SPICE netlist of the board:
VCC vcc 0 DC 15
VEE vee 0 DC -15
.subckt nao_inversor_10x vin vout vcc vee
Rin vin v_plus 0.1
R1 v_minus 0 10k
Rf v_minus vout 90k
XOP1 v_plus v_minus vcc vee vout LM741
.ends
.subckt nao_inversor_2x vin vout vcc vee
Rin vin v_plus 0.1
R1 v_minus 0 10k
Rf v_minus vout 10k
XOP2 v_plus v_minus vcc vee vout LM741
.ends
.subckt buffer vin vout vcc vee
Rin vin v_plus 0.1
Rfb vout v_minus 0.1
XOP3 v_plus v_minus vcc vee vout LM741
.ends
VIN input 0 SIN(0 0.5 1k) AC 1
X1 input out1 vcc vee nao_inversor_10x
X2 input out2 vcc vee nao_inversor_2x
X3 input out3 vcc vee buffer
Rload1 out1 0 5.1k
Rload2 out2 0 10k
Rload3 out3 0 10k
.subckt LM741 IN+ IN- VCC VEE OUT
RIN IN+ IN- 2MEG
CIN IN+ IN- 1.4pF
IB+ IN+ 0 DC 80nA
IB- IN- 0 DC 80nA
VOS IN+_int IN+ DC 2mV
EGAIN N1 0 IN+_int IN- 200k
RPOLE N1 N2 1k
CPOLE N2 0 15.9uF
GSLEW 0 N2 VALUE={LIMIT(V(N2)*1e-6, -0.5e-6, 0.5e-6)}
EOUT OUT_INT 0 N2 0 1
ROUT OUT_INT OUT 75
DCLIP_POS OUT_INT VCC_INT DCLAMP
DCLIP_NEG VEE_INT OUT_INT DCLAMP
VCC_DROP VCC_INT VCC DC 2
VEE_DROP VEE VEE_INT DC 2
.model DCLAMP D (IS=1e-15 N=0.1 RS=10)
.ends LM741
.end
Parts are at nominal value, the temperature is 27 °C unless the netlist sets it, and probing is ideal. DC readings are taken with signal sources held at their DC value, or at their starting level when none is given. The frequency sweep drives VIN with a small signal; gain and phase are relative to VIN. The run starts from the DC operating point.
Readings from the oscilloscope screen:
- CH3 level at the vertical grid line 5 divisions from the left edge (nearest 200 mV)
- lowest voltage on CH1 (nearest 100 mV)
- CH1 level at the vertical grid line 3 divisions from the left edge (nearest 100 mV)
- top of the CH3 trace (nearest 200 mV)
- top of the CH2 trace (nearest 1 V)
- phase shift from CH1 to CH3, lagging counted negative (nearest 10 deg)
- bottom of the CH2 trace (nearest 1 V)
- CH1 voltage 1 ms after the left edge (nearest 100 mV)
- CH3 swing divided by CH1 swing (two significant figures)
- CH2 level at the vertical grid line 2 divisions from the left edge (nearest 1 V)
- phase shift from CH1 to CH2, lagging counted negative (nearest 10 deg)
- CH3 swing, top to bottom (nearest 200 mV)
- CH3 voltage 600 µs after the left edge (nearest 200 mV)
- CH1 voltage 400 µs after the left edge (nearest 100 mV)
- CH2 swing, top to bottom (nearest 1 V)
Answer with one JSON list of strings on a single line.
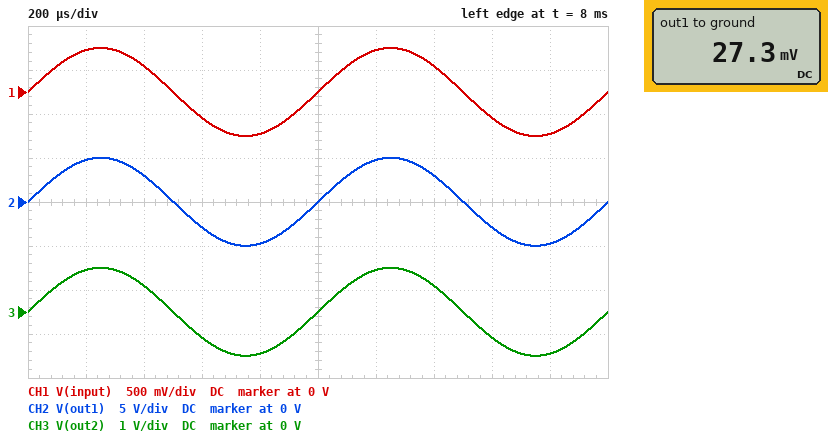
["0 V", "-500 mV", "-300 mV", "1.0 V", "5 V", "0 deg", "-5 V", "0 V", "2.0", "3 V", "0 deg", "2.0 V", "-600 mV", "300 mV", "10 V"]
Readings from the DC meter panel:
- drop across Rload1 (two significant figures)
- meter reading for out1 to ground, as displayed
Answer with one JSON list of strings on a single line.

["27 mV", "27.3 mV"]
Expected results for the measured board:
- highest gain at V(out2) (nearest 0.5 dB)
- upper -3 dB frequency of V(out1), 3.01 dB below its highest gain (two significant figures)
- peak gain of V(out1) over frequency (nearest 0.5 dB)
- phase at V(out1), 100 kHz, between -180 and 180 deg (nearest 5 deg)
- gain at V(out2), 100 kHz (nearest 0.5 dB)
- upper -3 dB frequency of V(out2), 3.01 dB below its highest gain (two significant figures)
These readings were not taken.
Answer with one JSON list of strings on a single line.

["6.0 dB", "200 kHz", "20.0 dB", "-25 deg", "6.0 dB", "1.0 MHz"]
